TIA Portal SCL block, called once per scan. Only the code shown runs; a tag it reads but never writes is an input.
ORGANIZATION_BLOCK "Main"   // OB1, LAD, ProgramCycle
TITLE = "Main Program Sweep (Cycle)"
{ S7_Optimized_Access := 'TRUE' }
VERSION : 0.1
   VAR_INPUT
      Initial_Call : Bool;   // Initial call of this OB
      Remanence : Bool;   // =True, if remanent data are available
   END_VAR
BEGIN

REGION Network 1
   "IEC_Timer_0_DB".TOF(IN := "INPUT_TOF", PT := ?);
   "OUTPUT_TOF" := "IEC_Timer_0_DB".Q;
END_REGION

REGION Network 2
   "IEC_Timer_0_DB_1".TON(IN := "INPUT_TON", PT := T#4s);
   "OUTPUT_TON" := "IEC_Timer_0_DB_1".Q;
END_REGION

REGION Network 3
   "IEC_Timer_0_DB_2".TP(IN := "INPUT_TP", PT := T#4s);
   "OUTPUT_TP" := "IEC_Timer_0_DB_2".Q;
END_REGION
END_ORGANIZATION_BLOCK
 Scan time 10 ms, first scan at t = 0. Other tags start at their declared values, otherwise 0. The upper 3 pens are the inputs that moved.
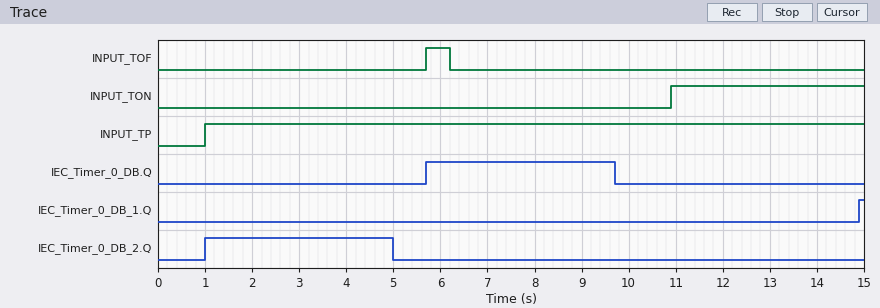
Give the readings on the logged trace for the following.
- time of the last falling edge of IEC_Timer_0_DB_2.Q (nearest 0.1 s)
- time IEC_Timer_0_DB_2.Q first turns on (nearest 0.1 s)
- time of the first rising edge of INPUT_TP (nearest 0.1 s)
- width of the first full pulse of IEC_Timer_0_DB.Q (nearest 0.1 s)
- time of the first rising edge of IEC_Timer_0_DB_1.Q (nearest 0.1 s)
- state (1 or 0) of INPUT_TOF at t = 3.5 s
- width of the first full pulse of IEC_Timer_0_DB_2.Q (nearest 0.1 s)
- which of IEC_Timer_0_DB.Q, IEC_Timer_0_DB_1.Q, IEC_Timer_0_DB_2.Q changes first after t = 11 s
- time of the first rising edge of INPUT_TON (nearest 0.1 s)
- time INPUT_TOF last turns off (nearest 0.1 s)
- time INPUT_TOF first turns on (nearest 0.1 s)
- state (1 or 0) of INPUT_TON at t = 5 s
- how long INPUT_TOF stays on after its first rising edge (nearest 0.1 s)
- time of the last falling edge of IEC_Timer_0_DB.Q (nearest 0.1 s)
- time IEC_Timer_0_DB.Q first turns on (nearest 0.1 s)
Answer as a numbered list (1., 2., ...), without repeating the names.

1. 5.0 s
2. 1.0 s
3. 1.0 s
4. 4.0 s
5. 14.9 s
6. 0
7. 4.0 s
8. IEC_Timer_0_DB_1.Q
9. 10.9 s
10. 6.2 s
11. 5.7 s
12. 0
13. 0.5 s
14. 9.7 s
15. 5.7 s
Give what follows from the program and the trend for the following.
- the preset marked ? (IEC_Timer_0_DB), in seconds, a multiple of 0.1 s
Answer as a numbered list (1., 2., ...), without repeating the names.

1. 3.5 s
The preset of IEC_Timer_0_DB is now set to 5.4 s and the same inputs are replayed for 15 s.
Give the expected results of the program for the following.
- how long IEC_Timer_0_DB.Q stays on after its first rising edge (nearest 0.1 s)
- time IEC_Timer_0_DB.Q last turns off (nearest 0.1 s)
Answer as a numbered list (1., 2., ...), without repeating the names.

1. 5.9 s
2. 11.6 s
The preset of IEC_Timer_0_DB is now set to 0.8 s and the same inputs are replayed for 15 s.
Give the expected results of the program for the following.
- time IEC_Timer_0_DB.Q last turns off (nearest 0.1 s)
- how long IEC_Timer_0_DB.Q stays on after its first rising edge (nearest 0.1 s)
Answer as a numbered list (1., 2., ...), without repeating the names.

1. 7.0 s
2. 1.3 s
